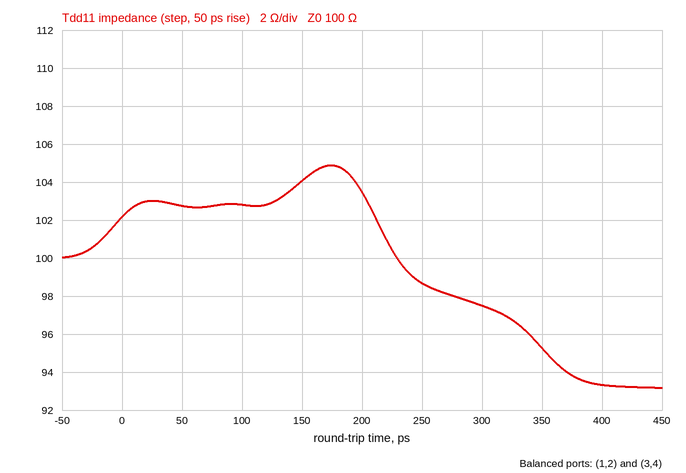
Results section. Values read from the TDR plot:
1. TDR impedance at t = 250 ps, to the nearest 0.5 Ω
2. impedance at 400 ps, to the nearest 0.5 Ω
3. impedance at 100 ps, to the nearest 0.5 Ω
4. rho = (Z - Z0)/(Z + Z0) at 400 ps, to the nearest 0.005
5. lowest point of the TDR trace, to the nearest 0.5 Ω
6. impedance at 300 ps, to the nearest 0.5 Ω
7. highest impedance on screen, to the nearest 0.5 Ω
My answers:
98.5 Ω
93.5 Ω
103.0 Ω
-0.035
93.0 Ω
97.5 Ω
105.0 Ω
